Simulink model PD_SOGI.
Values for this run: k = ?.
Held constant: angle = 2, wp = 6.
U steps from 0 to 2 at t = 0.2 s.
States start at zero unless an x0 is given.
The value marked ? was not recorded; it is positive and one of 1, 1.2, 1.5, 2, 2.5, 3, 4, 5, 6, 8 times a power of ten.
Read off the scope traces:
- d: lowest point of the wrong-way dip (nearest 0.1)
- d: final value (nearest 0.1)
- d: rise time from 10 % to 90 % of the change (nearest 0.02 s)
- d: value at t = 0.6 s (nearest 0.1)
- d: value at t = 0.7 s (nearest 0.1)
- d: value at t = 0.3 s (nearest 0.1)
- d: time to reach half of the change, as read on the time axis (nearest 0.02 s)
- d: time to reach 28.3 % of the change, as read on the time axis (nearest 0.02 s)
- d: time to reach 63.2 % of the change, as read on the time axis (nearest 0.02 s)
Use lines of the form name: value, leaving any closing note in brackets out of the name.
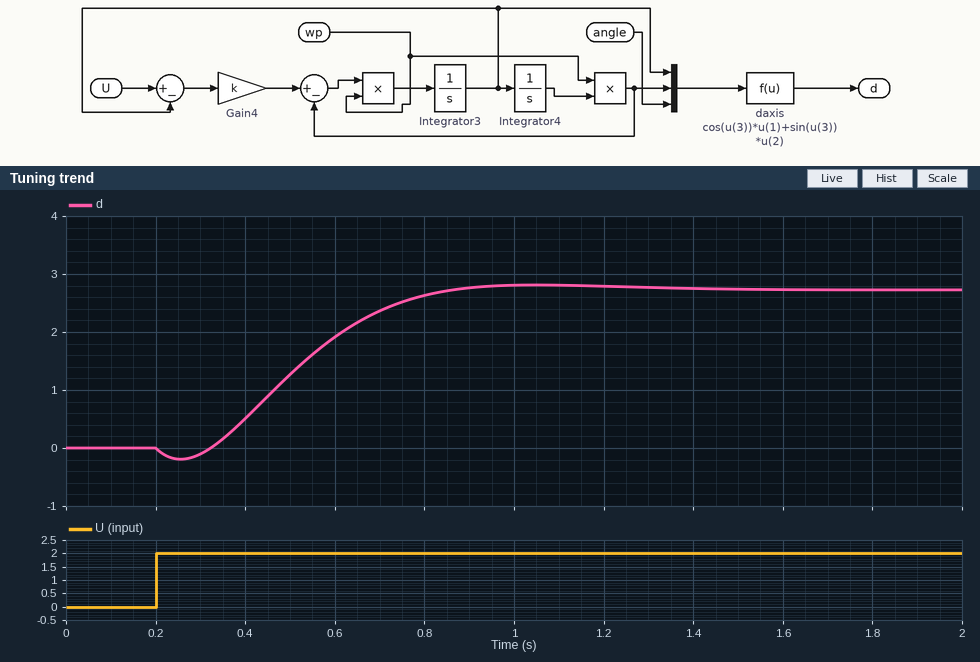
d: lowest point of the wrong-way dip: -0.2
d: final value: 2.7
d: rise time from 10 % to 90 % of the change: 0.36 s
d: value at t = 0.6 s: 1.9
d: value at t = 0.7 s: 2.4
d: value at t = 0.3 s: -0.1
d: time to reach half of the change, as read on the time axis: 0.52 s
d: time to reach 28.3 % of the change, as read on the time axis: 0.44 s
d: time to reach 63.2 % of the change, as read on the time axis: 0.56 s
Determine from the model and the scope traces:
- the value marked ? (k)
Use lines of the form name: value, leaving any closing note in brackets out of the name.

the value marked ?: 1.5
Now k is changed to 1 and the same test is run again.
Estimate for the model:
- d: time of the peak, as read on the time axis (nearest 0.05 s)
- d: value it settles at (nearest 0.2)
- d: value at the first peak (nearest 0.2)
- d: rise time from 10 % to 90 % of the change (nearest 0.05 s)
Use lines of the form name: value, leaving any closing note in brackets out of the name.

d: time of the peak, as read on the time axis: 0.85 s
d: value it settles at: 1.8
d: value at the first peak: 2.2
d: rise time from 10 % to 90 % of the change: 0.25 s
